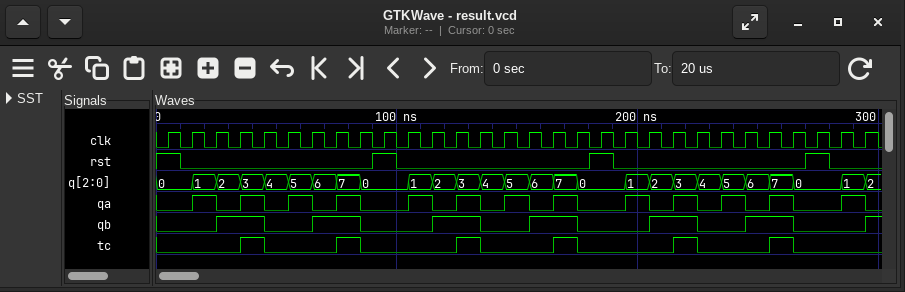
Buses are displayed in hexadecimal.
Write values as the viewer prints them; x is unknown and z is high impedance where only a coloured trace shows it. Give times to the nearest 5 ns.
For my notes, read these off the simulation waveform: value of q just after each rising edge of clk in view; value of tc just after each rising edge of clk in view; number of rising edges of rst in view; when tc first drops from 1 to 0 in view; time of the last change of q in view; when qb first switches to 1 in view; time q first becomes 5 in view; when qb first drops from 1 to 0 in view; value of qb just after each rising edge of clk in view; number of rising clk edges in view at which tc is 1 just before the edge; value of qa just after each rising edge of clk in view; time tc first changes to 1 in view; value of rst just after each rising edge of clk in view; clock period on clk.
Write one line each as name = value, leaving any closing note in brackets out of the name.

value of q just after each rising edge of clk in view = 0, 1, 2, 3, 4, 5, 6, 7, 0, 0, 1, 2, 3, 4, 5, 6, 7, 0, 0, 1, 2, 3, 4, 5, 6, 7, 0, 0, 1, 2
value of tc just after each rising edge of clk in view = 0 0 0 1 0 0 0 1 0 0 0 0 1 0 0 0 1 0 0 0 0 1 0 0 0 1 0 0 0 0
number of rising edges of rst in view = 3
when tc first drops from 1 to 0 in view = 45 ns
time of the last change of q in view = 295 ns
when qb first switches to 1 in view = 25 ns
time q first becomes 5 in view = 55 ns
when qb first drops from 1 to 0 in view = 45 ns
value of qb just after each rising edge of clk in view = 0 0 1 1 0 0 1 1 0 0 0 1 1 0 0 1 1 0 0 0 1 1 0 0 1 1 0 0 0 1
number of rising clk edges in view at which tc is 1 just before the edge = 6
value of qa just after each rising edge of clk in view = 0 1 0 1 0 1 0 1 0 0 1 0 1 0 1 0 1 0 0 1 0 1 0 1 0 1 0 0 1 0
time tc first changes to 1 in view = 35 ns
value of rst just after each rising edge of clk in view = 1 0 0 0 0 0 0 0 0 1 0 0 0 0 0 0 0 0 1 0 0 0 0 0 0 0 0 1 0 0
clock period on clk = 10 ns
